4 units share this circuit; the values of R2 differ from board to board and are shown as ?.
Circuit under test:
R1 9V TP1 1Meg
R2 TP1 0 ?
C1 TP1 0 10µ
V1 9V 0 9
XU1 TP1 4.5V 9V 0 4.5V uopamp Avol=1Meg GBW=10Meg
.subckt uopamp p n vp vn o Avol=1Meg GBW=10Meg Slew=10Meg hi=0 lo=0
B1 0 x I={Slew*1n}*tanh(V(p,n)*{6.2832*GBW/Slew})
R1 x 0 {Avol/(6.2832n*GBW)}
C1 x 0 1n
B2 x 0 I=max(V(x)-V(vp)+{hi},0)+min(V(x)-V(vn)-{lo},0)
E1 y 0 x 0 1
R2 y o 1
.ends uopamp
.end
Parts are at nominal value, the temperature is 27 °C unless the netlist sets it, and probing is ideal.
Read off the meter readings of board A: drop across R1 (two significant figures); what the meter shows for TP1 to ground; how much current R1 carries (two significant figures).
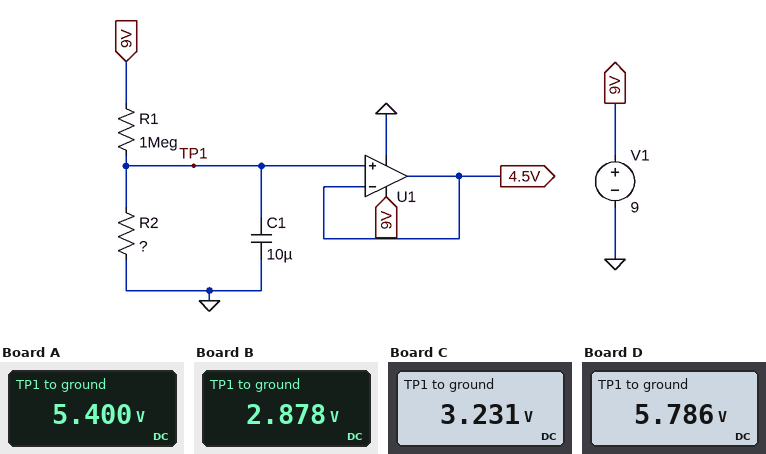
3.6 V
5.400 V
3.6 µA
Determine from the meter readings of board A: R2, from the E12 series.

1.5 MΩ
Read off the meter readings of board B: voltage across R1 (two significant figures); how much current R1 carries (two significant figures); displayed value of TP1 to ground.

6.1 V
6.1 µA
2.878 V
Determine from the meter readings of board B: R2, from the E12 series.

470 kΩ
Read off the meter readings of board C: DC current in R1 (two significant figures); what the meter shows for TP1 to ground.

5.8 µA
3.231 V
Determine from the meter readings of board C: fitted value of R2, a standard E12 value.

560 kΩ
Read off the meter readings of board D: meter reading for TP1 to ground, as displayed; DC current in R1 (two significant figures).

5.786 V
3.2 µA
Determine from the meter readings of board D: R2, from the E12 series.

1.8 MΩ
